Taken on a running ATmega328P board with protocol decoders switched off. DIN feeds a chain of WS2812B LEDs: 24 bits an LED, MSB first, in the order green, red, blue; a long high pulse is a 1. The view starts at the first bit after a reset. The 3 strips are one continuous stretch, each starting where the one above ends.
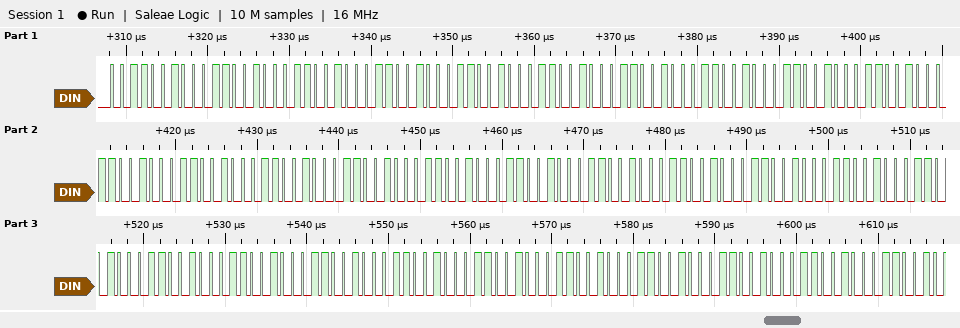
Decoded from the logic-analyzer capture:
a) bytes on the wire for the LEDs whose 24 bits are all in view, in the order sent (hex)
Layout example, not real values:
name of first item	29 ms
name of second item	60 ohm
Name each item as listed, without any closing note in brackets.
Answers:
bytes on the wire for the LEDs whose 24 bits are all in view, in the order sent	32 32 32 32 32 32 32 32 32 32 32 32 32 32 32 32 32 32 32 32 32 32 32 32 32 32 32 32 32 32
